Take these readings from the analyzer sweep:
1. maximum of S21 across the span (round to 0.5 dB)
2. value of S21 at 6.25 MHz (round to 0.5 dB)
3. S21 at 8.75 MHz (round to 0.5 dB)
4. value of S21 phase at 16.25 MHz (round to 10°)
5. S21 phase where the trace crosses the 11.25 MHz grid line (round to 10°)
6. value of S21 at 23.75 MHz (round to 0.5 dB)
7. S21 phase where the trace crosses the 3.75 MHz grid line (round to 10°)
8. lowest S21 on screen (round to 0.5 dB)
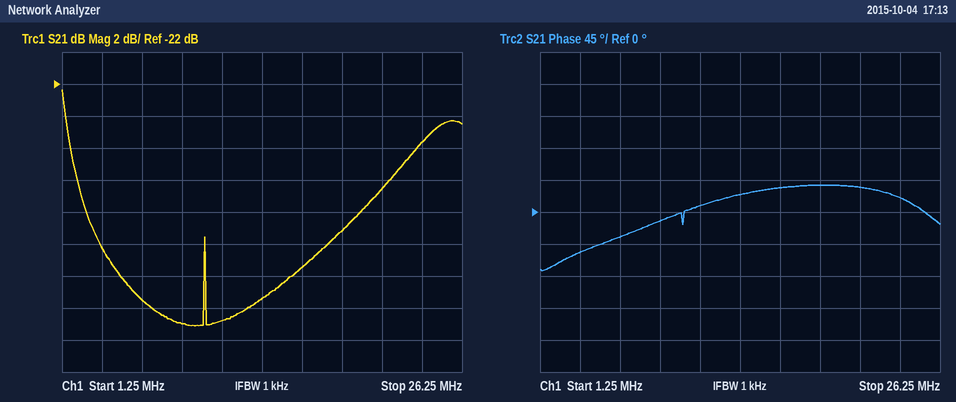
-22.5 dB
-35.5 dB
-37.0 dB
30°
10°
-25.5 dB
-60°
-37.0 dB
